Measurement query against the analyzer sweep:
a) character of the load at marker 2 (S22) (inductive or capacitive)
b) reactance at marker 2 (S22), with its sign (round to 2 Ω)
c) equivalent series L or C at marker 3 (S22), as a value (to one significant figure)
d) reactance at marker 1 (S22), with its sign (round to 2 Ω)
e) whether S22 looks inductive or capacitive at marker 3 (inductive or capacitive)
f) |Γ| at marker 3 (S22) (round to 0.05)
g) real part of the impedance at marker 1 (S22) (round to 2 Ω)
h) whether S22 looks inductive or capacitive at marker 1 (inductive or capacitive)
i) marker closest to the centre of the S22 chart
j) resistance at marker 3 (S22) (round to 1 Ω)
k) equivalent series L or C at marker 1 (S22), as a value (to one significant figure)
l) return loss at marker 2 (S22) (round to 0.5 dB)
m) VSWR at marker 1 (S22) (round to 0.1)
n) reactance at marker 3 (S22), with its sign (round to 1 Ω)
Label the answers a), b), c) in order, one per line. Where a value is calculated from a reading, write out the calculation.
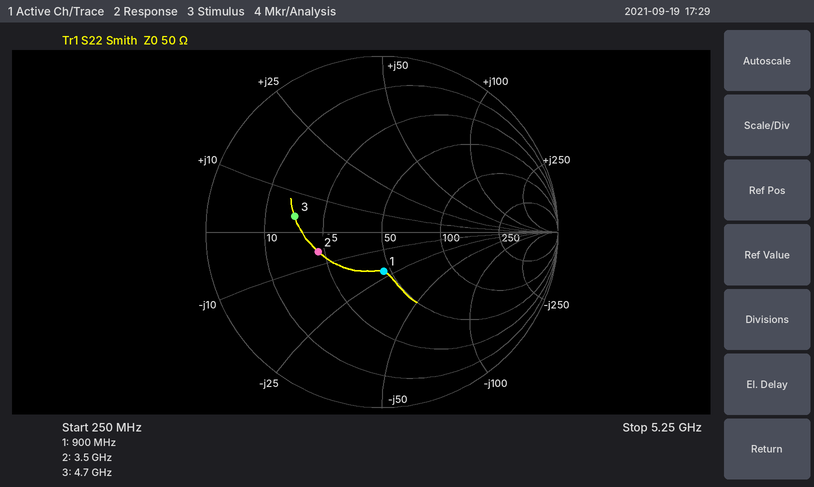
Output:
a) capacitive
b) -6 Ω
c) L = 4 Ω/(2π × 4.7 GHz) ≈ 135 pH, so 100 pH to one significant figure
d) -22 Ω
e) inductive
f) 0.50
g) 46 Ω
h) capacitive
i) marker 1
j) 17 Ω
k) C = 1/(2π × 900 MHz × 22 Ω) ≈ 8 pF
l) 8.5 dB
m) 1.6
n) +4 Ω
